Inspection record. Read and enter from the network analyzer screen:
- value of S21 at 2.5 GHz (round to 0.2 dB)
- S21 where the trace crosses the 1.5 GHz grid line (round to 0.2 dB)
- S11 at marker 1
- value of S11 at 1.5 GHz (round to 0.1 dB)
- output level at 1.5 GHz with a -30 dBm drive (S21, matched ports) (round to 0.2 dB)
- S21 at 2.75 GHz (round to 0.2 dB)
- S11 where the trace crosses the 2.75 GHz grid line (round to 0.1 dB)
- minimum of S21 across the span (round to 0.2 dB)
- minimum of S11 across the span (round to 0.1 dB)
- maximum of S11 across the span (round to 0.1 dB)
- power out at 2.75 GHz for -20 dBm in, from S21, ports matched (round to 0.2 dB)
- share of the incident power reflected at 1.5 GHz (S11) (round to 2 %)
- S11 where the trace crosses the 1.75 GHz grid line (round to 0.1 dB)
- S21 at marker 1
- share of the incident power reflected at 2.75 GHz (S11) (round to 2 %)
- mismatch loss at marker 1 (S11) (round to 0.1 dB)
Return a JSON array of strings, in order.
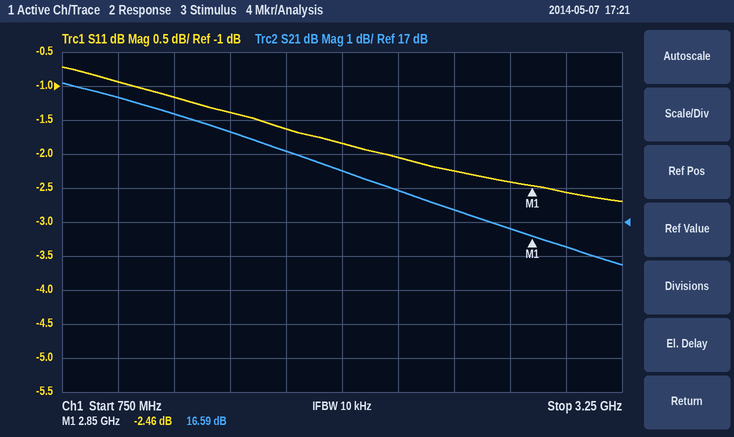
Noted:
["17.4 dB", "19.6 dB", "-2.46 dB", "-1.4 dB", "-10.4 dBm", "16.8 dB", "-2.4 dB", "15.8 dB", "-2.7 dB", "-0.7 dB", "-3.2 dBm", "72 %", "-1.6 dB", "16.59 dB", "58 %", "3.6 dB"]
